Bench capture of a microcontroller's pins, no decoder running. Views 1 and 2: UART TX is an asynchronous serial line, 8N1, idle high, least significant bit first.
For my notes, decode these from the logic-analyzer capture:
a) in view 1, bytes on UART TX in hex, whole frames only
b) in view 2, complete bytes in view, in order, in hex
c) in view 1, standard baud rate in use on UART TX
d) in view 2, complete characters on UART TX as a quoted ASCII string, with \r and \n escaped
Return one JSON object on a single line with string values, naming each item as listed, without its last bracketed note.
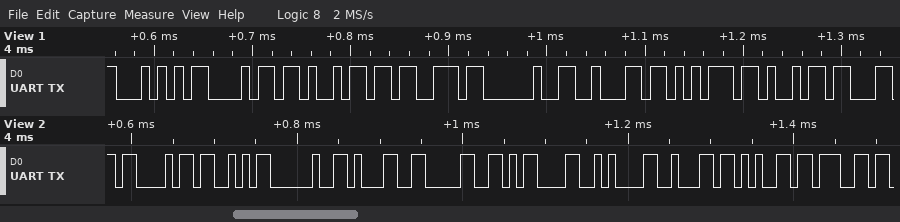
{"in view 1, bytes on UART TX in hex, whole frames only": "54 68 69 73 20 62 75 69", "in view 2, complete bytes in view, in order, in hex": "43 53 20 31 30 0D 0A 62 65 67", "in view 1, standard baud rate in use on UART TX": "115200 baud", "in view 2, complete characters on UART TX as a quoted ASCII string, with \\r and \\n escaped": "\"CS 10\\r\\nbeg\""}
